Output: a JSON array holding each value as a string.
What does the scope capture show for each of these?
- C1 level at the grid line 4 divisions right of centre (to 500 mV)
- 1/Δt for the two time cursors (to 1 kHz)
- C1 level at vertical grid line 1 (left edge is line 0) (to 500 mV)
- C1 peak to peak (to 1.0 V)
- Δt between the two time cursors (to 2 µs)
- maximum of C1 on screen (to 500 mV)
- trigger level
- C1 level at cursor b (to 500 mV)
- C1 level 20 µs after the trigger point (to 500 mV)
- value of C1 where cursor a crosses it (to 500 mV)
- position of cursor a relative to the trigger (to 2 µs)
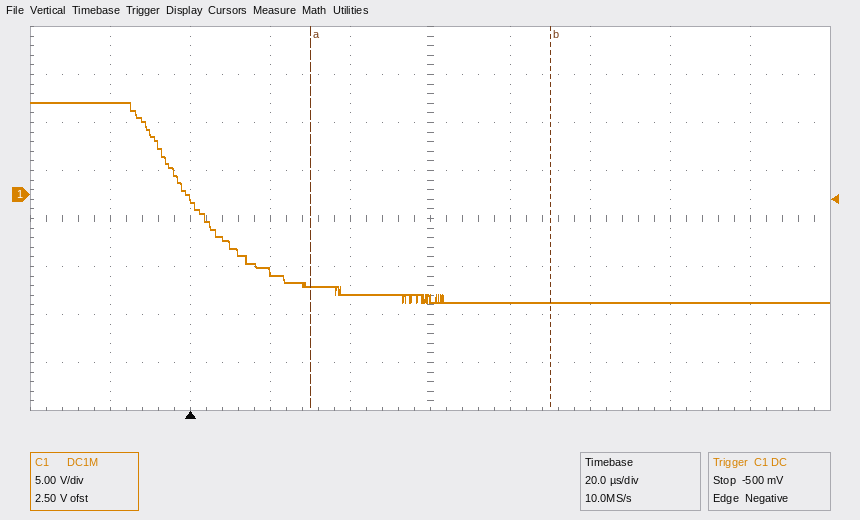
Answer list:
["-11.0 V", "17 kHz", "9.5 V", "21.0 V", "60 µs", "9.5 V", "-500 mV", "-11.0 V", "-8.0 V", "-9.5 V", "+30 µs"]
